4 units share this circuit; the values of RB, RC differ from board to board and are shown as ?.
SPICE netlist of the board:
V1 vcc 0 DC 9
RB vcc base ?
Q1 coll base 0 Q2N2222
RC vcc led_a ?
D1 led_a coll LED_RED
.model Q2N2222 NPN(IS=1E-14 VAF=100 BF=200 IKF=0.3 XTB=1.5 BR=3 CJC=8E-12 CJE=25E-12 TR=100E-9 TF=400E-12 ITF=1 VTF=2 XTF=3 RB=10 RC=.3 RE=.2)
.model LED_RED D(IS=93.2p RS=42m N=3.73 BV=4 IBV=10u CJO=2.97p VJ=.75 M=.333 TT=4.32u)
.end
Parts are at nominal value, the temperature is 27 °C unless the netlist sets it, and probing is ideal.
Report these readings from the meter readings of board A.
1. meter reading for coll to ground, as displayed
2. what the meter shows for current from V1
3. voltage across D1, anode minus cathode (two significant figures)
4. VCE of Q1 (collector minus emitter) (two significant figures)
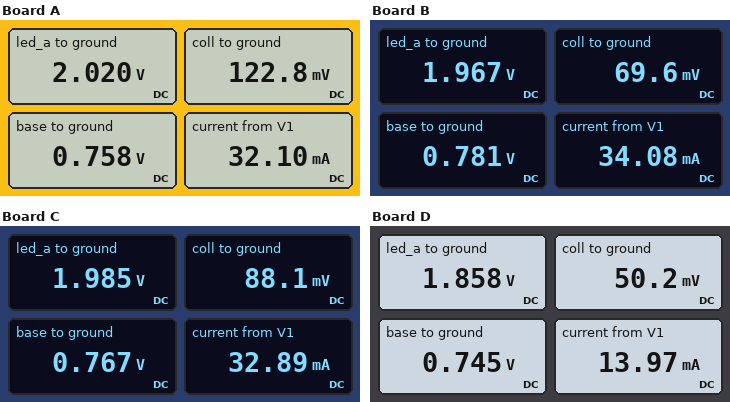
122.8 mV
32.10 mA
1.9 V
120 mV
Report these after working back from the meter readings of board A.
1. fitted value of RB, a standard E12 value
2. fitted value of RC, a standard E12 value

22 kΩ
220 Ω
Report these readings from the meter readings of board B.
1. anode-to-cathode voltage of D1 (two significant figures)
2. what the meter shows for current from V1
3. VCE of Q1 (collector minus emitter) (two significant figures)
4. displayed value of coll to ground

1.9 V
34.08 mA
70 mV
69.6 mV
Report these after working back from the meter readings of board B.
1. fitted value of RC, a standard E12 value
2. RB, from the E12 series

220 Ω
3.9 kΩ
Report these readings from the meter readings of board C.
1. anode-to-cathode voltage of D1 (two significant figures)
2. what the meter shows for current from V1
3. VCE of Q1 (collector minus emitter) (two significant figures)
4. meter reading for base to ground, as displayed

1.9 V
32.89 mA
88 mV
0.767 V
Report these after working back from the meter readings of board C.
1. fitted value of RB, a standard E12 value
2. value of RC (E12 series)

8.2 kΩ
220 Ω
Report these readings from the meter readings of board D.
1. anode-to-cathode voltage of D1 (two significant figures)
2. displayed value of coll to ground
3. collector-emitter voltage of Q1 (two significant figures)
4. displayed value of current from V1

1.8 V
50.2 mV
50 mV
13.97 mA
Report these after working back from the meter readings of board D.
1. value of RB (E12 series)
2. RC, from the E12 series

6.8 kΩ
560 Ω
